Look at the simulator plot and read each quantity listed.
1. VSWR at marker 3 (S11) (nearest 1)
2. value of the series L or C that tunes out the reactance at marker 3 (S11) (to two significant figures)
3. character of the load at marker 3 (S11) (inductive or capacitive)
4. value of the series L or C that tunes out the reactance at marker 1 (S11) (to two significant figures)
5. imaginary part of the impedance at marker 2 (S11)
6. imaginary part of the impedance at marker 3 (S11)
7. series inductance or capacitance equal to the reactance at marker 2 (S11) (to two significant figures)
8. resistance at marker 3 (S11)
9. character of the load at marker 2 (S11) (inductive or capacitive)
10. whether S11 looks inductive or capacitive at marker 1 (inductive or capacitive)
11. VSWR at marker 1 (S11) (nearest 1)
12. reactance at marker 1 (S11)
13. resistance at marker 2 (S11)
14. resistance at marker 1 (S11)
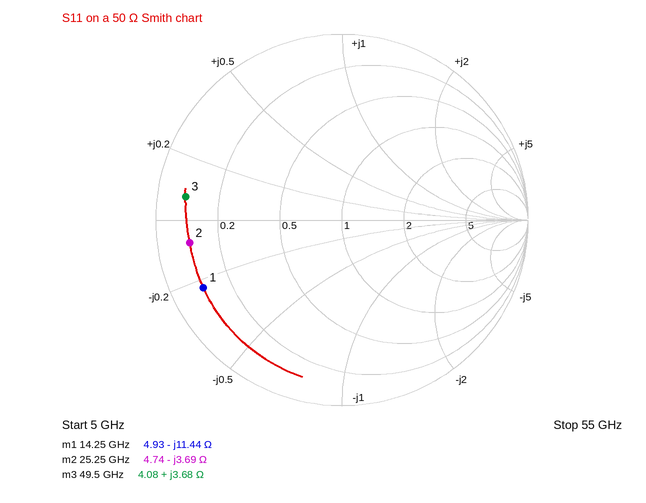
12
870 fF
inductive
130 pH
-3.69 Ω
+3.68 Ω
1.7 pF
4.08 Ω
capacitive
capacitive
11
-11.44 Ω
4.74 Ω
4.93 Ω
